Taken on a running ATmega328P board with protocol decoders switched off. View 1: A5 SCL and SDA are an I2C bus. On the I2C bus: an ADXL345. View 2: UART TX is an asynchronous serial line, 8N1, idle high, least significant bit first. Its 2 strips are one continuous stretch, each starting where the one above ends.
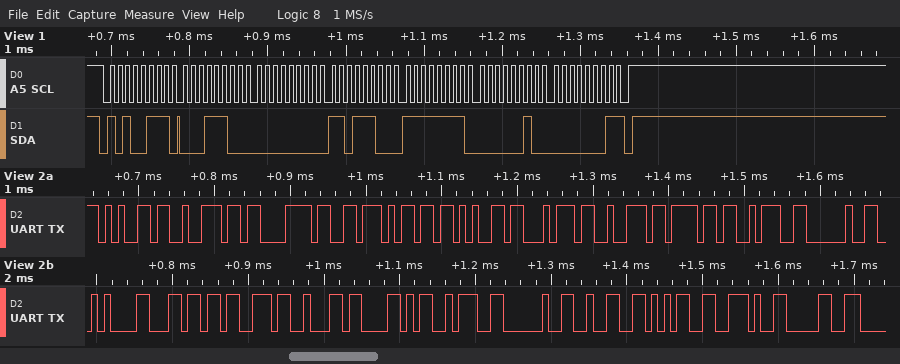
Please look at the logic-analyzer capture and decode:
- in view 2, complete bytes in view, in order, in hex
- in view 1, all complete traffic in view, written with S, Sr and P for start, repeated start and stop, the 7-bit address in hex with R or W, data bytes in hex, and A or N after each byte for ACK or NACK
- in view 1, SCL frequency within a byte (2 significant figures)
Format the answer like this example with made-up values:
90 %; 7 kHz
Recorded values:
0x65 0x72 0xC3 0xB3 0x6D 0x65 0x74 0x72 0x6F 0x3A 0x20 0x0A 0x6C 0x73 0x62 0x58 0x3A 0x20 0x32 0x35 0x2E 0x30; S 53R A 1C A 00 A DC A FF A 02 A 01 N P; 100 kHz
